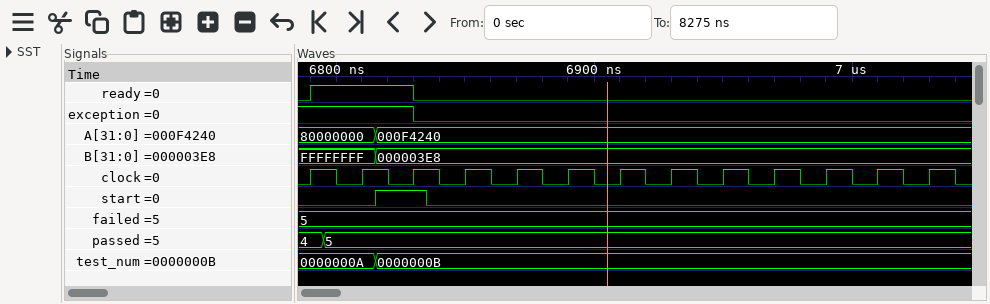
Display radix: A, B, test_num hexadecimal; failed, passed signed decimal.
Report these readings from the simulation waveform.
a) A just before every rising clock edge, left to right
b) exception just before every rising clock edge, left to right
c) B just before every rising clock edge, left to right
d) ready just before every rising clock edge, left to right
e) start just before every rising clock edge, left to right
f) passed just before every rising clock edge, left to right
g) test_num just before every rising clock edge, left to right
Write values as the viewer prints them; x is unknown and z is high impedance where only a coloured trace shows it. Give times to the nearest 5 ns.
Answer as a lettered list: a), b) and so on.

a) 80000000, 80000000, 000F4240, 000F4240, 000F4240, 000F4240, 000F4240, 000F4240, 000F4240, 000F4240, 000F4240, 000F4240, 000F4240
b) 1 1 1 0 0 0 0 0 0 0 0 0 0
c) FFFFFFFF, FFFFFFFF, 000003E8, 000003E8, 000003E8, 000003E8, 000003E8, 000003E8, 000003E8, 000003E8, 000003E8, 000003E8, 000003E8
d) 0 1 1 0 0 0 0 0 0 0 0 0 0
e) 0 0 1 0 0 0 0 0 0 0 0 0 0
f) 4, 5, 5, 5, 5, 5, 5, 5, 5, 5, 5, 5, 5
g) 0000000A, 0000000A, 0000000B, 0000000B, 0000000B, 0000000B, 0000000B, 0000000B, 0000000B, 0000000B, 0000000B, 0000000B, 0000000B
